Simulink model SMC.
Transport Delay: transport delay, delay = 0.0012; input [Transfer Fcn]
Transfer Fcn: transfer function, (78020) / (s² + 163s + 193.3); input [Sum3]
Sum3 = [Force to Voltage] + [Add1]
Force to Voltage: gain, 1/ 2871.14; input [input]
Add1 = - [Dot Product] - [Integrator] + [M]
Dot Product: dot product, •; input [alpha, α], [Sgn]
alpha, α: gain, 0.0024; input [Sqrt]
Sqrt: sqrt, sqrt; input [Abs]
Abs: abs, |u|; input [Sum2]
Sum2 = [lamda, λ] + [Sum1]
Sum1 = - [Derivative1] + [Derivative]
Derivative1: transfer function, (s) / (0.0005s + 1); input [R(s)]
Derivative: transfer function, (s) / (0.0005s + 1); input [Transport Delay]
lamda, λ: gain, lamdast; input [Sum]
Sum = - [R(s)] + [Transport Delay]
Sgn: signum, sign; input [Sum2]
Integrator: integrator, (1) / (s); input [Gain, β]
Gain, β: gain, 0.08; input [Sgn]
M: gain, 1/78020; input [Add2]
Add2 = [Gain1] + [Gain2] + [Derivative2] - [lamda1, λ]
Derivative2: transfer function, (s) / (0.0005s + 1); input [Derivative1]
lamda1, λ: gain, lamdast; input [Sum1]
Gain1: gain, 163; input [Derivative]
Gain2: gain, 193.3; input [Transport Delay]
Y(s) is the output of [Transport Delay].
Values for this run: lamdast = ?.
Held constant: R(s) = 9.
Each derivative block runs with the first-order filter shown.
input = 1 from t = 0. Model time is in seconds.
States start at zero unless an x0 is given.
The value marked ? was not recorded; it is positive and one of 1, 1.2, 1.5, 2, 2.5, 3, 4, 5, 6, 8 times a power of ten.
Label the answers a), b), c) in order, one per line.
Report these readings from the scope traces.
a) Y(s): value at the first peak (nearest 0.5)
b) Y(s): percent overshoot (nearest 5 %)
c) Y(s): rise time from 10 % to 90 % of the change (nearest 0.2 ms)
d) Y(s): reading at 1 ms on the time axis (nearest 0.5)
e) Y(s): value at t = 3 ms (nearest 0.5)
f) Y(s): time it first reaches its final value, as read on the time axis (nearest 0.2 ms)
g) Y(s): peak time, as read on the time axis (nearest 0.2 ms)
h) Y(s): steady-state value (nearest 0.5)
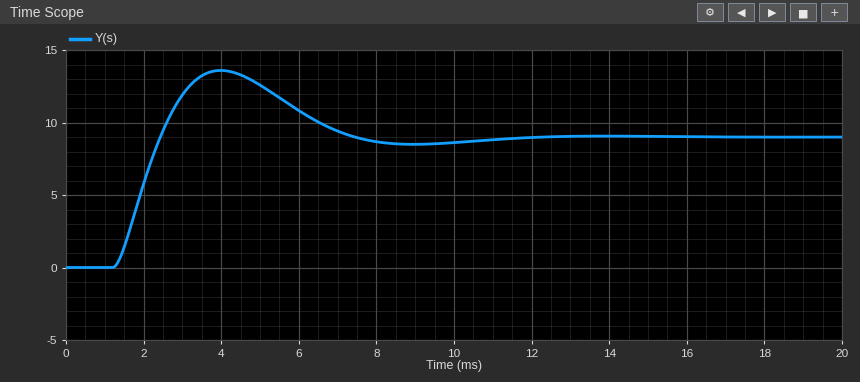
a) 13.5
b) 50 %
c) 0.8 ms
d) 0.0
e) 12.0
f) 2.4 ms
g) 4.0 ms
h) 9.0
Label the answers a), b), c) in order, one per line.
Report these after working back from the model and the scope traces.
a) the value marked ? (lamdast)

a) 500
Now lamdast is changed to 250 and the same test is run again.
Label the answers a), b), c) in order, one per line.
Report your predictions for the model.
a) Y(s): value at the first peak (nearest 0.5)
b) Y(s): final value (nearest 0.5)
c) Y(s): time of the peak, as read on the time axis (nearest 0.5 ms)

a) 10.5
b) 9.0
c) 4.5 ms
